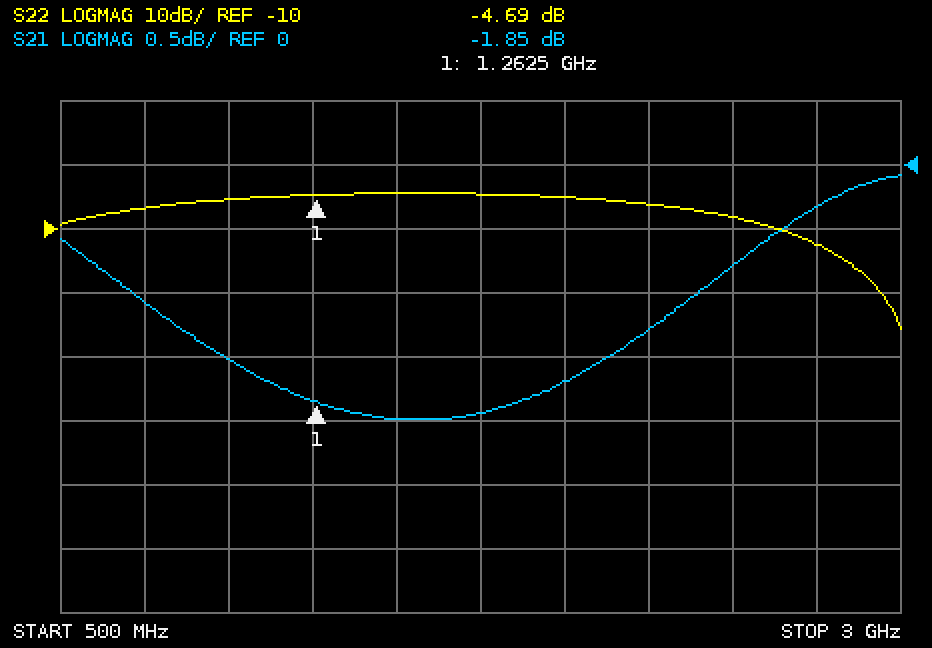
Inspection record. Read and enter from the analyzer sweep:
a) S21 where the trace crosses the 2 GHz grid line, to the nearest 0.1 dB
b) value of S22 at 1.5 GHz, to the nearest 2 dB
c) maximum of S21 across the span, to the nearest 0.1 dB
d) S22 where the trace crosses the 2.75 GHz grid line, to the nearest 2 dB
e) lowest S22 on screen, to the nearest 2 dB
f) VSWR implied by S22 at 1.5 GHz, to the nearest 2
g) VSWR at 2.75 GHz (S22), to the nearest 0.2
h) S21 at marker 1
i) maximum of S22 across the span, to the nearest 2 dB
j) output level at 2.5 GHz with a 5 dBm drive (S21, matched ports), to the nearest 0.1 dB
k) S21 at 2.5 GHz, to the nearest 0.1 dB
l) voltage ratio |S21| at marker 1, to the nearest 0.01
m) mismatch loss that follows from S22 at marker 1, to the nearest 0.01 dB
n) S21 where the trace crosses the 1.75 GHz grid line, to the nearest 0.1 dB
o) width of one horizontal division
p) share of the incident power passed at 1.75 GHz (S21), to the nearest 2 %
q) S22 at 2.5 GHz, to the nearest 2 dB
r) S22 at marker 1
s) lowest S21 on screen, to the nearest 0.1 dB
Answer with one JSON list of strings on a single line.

["-1.7 dB", "-4 dB", "-0.1 dB", "-12 dB", "-26 dB", "4", "1.6", "-1.85 dB", "-4 dB", "4.2 dBm", "-0.8 dB", "0.81", "1.80 dB", "-1.9 dB", "250 MHz", "64 %", "-8 dB", "-4.69 dB", "-2.0 dB"]
